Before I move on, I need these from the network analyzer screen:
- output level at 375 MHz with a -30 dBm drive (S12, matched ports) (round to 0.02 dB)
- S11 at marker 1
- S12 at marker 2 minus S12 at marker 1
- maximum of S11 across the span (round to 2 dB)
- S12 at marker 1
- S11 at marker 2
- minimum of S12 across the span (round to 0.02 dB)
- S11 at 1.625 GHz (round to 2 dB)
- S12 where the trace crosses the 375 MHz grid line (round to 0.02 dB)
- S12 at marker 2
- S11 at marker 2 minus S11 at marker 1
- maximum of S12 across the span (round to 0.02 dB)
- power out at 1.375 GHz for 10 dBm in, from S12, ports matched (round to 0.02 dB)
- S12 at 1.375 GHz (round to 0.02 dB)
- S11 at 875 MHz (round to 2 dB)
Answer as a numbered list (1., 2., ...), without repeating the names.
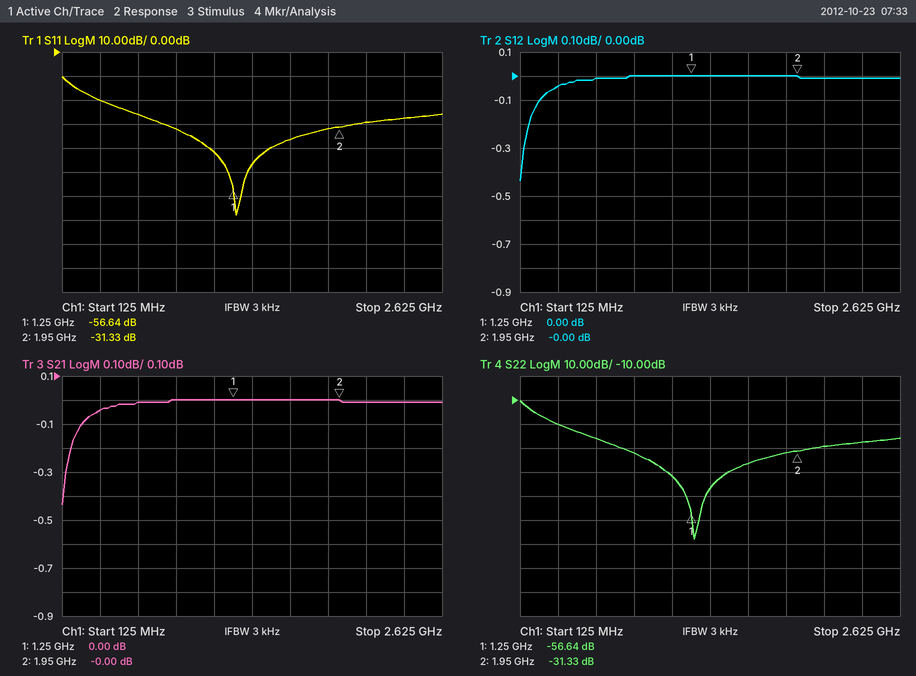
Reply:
1. -30.04 dBm
2. -56.64 dB
3. 0.00 dB
4. -10 dB
5. 0.00 dB
6. -31.33 dB
7. -0.44 dB
8. -36 dB
9. -0.04 dB
10. -0.00 dB
11. 25.31 dB
12. 0.00 dB
13. 10.00 dBm
14. 0.00 dB
15. -32 dB
